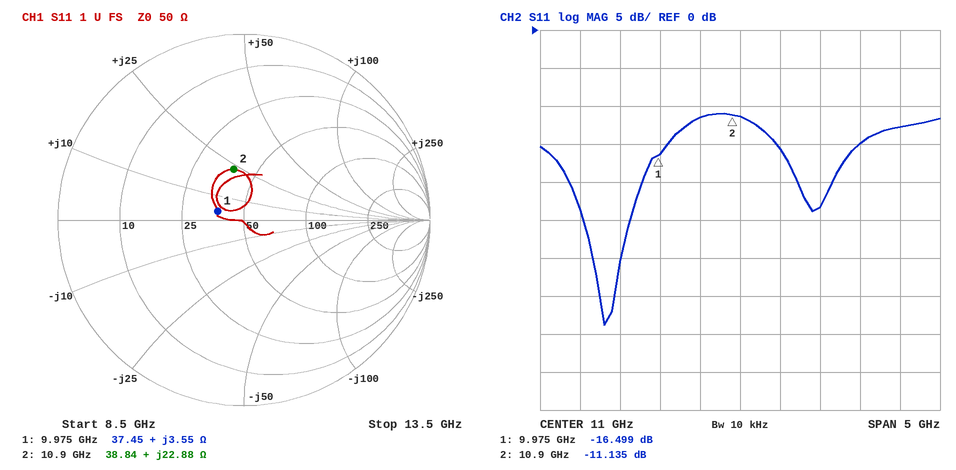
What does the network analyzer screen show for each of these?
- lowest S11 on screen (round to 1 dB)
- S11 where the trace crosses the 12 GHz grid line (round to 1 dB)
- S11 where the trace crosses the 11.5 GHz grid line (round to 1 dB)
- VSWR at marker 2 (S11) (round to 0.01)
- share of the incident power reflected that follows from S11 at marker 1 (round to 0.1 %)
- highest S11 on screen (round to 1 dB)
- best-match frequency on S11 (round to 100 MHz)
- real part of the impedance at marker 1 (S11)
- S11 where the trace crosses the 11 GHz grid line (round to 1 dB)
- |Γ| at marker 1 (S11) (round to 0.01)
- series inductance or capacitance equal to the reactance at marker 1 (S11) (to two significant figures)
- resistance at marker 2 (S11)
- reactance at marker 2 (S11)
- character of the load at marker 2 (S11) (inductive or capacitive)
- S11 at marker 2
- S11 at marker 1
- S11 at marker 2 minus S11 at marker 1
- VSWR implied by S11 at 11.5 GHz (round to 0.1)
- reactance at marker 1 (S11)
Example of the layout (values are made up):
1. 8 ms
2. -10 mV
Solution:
1. -39 dB
2. -23 dB
3. -16 dB
4. 1.77
5. 2.2 %
6. -11 dB
7. 9.3 GHz
8. 37.45 Ω
9. -11 dB
10. 0.15
11. 57 pH
12. 38.84 Ω
13. +22.88 Ω
14. inductive
15. -11.135 dB
16. -16.499 dB
17. 5.364 dB
18. 1.4
19. +3.55 Ω
